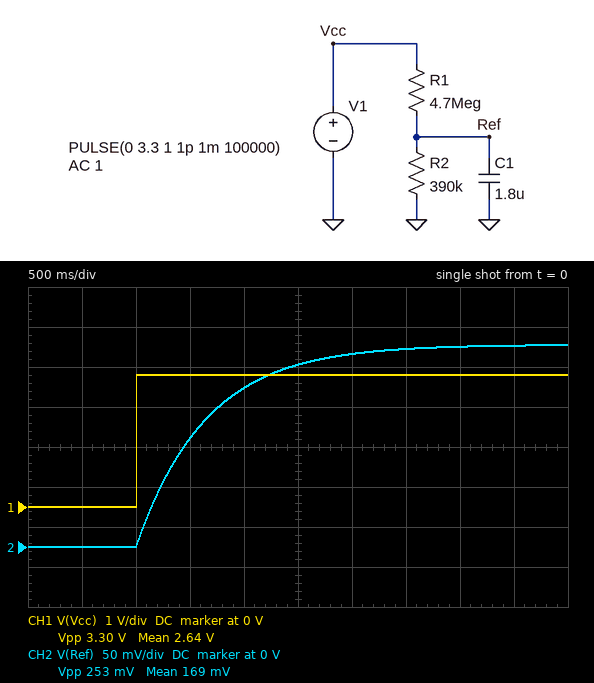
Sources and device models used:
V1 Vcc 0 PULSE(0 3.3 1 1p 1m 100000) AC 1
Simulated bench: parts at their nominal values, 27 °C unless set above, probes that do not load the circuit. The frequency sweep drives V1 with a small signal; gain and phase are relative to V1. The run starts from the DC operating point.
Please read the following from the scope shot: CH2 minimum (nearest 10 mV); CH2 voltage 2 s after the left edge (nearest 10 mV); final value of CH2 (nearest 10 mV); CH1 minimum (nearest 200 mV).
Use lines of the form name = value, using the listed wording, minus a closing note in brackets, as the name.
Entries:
CH2 minimum = 0 V
CH2 voltage 2 s after the left edge = 200 mV
final value of CH2 = 250 mV
CH1 minimum = 0 V
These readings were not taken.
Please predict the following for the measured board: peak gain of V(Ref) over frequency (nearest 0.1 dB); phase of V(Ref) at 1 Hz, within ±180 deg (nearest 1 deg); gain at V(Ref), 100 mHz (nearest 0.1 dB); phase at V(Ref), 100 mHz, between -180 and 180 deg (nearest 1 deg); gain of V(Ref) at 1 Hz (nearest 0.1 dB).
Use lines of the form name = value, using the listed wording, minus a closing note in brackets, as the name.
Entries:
peak gain of V(Ref) over frequency = -22.3 dB
phase of V(Ref) at 1 Hz, within ±180 deg = -76 deg
gain at V(Ref), 100 mHz = -23.0 dB
phase at V(Ref), 100 mHz, between -180 and 180 deg = -22 deg
gain of V(Ref) at 1 Hz = -34.8 dB
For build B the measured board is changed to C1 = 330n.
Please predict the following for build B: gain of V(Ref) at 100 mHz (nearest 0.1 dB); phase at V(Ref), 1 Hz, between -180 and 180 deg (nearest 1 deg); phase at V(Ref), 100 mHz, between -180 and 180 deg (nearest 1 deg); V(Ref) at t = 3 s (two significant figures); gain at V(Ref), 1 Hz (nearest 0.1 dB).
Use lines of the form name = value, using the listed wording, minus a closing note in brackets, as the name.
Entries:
gain of V(Ref) at 100 mHz = -22.3 dB
phase at V(Ref), 1 Hz, between -180 and 180 deg = -37 deg
phase at V(Ref), 100 mHz, between -180 and 180 deg = -4 deg
V(Ref) at t = 3 s = 250 mV
gain at V(Ref), 1 Hz = -24.2 dB
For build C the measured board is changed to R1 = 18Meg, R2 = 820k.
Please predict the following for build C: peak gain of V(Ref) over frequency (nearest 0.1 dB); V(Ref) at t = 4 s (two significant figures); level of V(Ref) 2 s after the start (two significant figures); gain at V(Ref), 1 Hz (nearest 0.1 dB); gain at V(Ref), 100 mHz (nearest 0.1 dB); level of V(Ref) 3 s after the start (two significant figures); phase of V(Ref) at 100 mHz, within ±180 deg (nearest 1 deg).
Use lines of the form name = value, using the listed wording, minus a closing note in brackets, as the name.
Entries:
peak gain of V(Ref) over frequency = -27.2 dB
V(Ref) at t = 4 s = 130 mV
level of V(Ref) 2 s after the start = 73 mV
gain at V(Ref), 1 Hz = -46.2 dB
gain at V(Ref), 100 mHz = -29.7 dB
level of V(Ref) 3 s after the start = 110 mV
phase of V(Ref) at 100 mHz, within ±180 deg = -42 deg
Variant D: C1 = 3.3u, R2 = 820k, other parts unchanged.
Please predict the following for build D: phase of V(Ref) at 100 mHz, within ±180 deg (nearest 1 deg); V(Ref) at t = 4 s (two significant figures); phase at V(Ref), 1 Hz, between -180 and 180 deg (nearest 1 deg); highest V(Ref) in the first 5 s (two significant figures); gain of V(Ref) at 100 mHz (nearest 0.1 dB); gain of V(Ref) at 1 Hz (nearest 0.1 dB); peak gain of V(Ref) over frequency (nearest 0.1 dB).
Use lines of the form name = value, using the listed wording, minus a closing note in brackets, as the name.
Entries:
phase of V(Ref) at 100 mHz, within ±180 deg = -55 deg
V(Ref) at t = 4 s = 360 mV
phase at V(Ref), 1 Hz, between -180 and 180 deg = -86 deg
highest V(Ref) in the first 5 s = 400 mV
gain of V(Ref) at 100 mHz = -21.5 dB
gain of V(Ref) at 1 Hz = -39.8 dB
peak gain of V(Ref) over frequency = -16.6 dB
